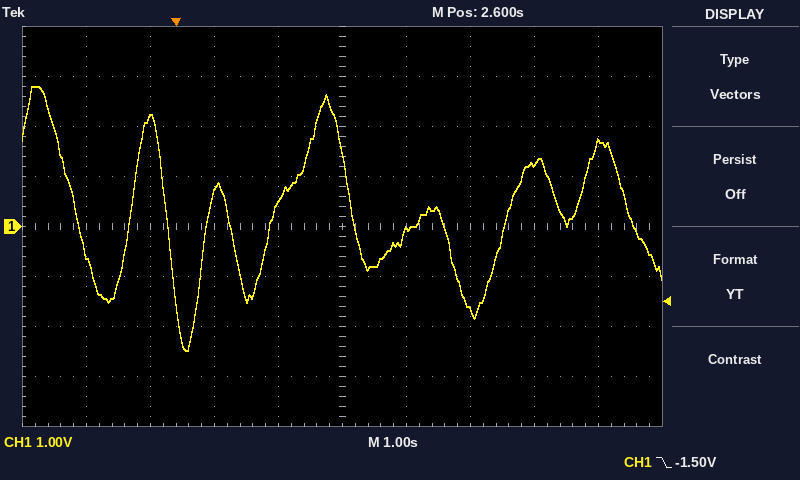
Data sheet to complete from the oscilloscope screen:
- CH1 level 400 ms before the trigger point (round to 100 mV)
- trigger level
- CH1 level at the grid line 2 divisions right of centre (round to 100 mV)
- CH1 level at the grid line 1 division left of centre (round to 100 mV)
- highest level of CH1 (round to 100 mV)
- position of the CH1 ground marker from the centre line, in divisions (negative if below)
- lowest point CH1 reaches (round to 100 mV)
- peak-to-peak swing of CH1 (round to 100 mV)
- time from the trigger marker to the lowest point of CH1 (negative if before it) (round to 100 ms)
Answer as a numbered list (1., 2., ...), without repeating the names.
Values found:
1. 2.2 V
2. -1.50 V
3. -1.7 V
4. 500 mV
5. 2.8 V
6. 0.0 div
7. -2.5 V
8. 5.3 V
9. +200 ms
